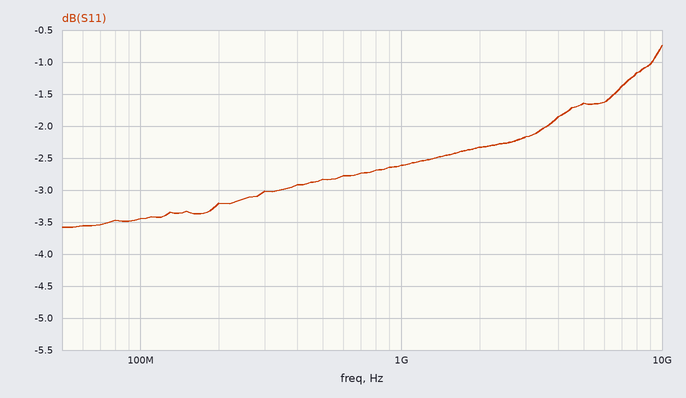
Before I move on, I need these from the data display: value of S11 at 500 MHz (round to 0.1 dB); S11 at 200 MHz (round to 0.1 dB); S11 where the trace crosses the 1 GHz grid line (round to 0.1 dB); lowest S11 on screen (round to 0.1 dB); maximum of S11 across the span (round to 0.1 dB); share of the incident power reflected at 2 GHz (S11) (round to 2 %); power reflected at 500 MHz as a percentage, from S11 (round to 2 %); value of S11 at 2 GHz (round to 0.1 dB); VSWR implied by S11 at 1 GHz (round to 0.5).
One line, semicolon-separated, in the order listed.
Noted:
-2.8 dB; -3.2 dB; -2.6 dB; -3.6 dB; -0.7 dB; 58 %; 52 %; -2.3 dB; 6.5
